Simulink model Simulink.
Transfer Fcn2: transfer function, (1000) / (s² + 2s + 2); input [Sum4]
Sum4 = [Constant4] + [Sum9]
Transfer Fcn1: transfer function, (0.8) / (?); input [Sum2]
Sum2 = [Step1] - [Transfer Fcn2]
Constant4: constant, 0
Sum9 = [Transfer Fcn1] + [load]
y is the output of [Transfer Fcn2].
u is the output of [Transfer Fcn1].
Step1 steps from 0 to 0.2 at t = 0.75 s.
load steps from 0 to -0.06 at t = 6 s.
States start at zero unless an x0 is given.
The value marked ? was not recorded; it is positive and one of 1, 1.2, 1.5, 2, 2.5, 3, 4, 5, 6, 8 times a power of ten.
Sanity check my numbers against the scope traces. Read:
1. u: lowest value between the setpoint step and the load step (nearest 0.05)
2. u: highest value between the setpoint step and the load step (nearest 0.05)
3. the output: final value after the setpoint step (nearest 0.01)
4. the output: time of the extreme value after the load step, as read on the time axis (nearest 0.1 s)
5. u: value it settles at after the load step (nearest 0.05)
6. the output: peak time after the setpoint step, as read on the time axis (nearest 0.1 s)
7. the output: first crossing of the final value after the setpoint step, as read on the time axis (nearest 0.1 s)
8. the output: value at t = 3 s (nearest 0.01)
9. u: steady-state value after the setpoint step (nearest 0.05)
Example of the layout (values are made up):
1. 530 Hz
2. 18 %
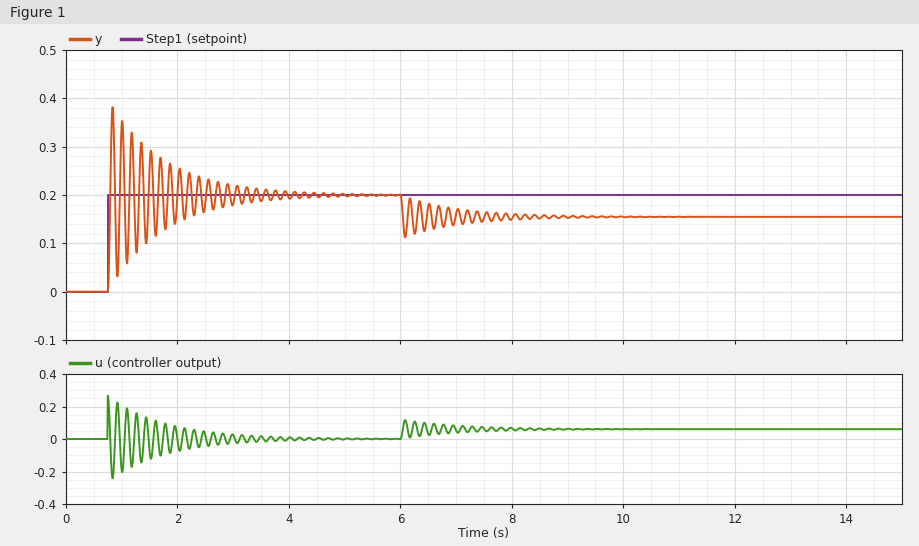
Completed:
1. -0.25
2. 0.25
3. 0.20
4. 6.1 s
5. 0.05
6. 0.8 s
7. 0.8 s
8. 0.18
9. 0.00
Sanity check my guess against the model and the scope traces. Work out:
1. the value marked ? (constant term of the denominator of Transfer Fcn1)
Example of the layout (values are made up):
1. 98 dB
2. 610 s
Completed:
1. 0.6
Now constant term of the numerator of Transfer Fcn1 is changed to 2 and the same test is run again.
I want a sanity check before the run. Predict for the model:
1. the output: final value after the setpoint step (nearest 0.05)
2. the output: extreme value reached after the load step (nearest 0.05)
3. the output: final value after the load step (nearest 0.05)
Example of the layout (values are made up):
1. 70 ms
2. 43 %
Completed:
1. 0.20
2. 0.15
3. 0.20
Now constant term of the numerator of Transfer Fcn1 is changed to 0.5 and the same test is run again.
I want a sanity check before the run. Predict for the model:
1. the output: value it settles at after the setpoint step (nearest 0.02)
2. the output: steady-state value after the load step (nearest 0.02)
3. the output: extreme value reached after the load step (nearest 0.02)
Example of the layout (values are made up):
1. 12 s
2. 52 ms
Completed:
1. 0.20
2. 0.12
3. 0.06
